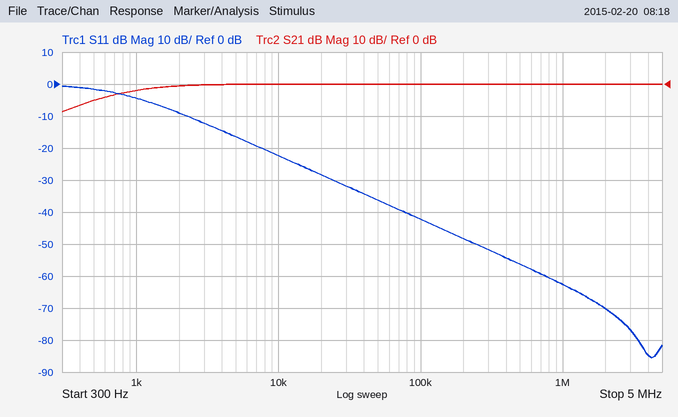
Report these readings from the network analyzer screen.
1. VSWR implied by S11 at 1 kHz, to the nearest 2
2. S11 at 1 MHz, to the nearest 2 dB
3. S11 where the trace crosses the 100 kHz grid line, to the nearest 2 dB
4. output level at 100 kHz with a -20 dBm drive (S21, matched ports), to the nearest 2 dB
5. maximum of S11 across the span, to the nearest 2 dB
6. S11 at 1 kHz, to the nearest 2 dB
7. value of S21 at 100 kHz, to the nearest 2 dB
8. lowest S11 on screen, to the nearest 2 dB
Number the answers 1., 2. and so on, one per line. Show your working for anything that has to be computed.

1. |Γ| = 10^(-4/20) = 0.6310; VSWR = (1 + 0.6310)/(1 − 0.6310) ≈ 4
2. -62 dB
3. -42 dB
4. -20 dBm + (0 dB) = -20 dBm
5. 0 dB
6. -4 dB
7. 0 dB
8. -86 dB
